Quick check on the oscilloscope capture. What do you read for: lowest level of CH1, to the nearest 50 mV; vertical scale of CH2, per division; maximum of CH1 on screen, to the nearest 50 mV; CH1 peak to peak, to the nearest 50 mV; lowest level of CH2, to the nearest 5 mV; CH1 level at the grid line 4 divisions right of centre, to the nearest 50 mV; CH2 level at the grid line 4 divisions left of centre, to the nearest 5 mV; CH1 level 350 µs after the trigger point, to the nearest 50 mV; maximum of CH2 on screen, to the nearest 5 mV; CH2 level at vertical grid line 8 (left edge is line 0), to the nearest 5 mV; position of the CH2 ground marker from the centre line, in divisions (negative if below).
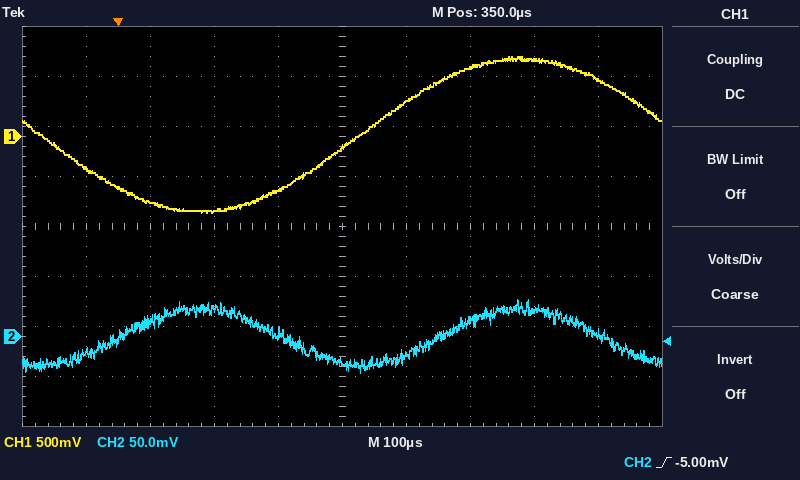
-750 mV
50 mV
800 mV
1.55 V
-35 mV
550 mV
-15 mV
-100 mV
35 mV
25 mV
-2.2 div
